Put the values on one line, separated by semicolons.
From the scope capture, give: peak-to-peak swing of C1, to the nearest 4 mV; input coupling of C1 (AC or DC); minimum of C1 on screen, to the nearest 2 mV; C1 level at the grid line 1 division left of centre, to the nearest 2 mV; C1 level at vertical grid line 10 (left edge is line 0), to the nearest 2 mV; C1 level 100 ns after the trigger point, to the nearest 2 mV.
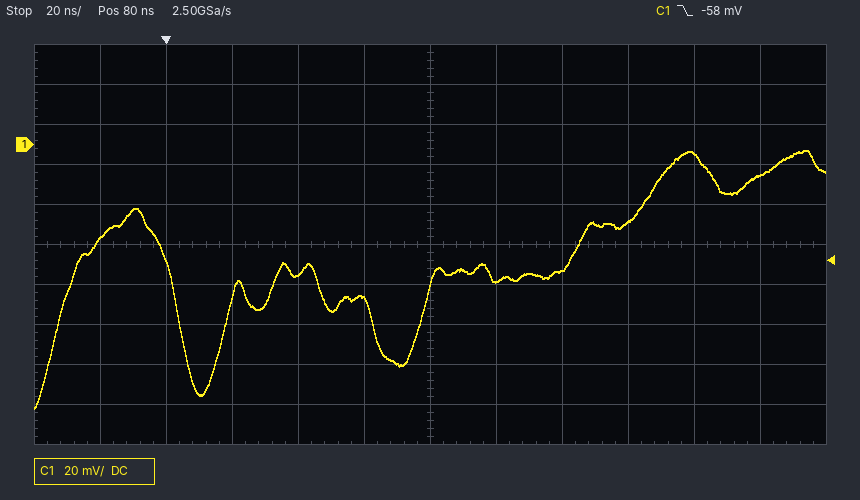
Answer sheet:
128 mV; DC; -132 mV; -78 mV; -4 mV; -68 mV
